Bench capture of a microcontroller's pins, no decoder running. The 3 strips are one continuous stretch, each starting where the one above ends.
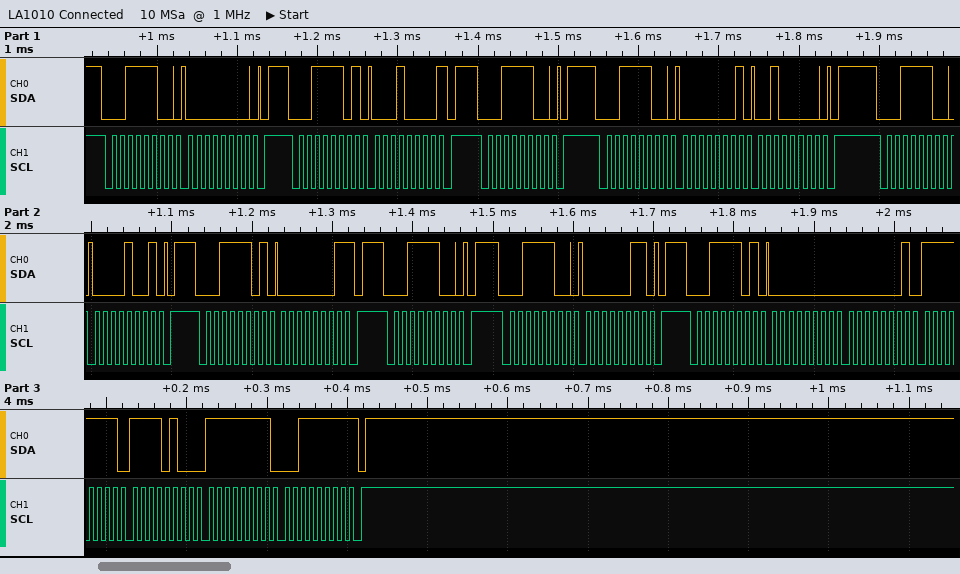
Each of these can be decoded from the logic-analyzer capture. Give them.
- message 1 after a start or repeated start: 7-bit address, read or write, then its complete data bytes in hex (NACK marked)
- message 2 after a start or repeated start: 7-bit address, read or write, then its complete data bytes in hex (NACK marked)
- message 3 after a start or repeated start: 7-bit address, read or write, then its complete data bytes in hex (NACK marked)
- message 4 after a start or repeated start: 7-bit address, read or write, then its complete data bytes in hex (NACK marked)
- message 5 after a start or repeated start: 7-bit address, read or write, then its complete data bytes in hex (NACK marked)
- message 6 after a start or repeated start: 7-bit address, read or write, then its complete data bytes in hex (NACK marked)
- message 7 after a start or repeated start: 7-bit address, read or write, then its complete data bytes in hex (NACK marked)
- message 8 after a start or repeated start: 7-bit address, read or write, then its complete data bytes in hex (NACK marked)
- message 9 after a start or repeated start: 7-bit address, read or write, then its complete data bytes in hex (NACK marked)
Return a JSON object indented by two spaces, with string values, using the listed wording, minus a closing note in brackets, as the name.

{
  "message 1 after a start or repeated start: 7-bit address, read or write, then its complete data bytes in hex": "0x1E write: 00",
  "message 2 after a start or repeated start: 7-bit address, read or write, then its complete data bytes in hex": "0x1E read: 10 NACK",
  "message 3 after a start or repeated start: 7-bit address, read or write, then its complete data bytes in hex": "0x1E write",
  "message 4 after a start or repeated start: 7-bit address, read or write, then its complete data bytes in hex": "0x1E write: 01 20",
  "message 5 after a start or repeated start: 7-bit address, read or write, then its complete data bytes in hex": "0x1E write: 09",
  "message 6 after a start or repeated start: 7-bit address, read or write, then its complete data bytes in hex": "0x1E read: 01 NACK",
  "message 7 after a start or repeated start: 7-bit address, read or write, then its complete data bytes in hex": "0x1E write",
  "message 8 after a start or repeated start: 7-bit address, read or write, then its complete data bytes in hex": "0x1E write: 03",
  "message 9 after a start or repeated start: 7-bit address, read or write, then its complete data bytes in hex": "0x1E read: 00 01 FF F4 FF 3F NACK"
}
